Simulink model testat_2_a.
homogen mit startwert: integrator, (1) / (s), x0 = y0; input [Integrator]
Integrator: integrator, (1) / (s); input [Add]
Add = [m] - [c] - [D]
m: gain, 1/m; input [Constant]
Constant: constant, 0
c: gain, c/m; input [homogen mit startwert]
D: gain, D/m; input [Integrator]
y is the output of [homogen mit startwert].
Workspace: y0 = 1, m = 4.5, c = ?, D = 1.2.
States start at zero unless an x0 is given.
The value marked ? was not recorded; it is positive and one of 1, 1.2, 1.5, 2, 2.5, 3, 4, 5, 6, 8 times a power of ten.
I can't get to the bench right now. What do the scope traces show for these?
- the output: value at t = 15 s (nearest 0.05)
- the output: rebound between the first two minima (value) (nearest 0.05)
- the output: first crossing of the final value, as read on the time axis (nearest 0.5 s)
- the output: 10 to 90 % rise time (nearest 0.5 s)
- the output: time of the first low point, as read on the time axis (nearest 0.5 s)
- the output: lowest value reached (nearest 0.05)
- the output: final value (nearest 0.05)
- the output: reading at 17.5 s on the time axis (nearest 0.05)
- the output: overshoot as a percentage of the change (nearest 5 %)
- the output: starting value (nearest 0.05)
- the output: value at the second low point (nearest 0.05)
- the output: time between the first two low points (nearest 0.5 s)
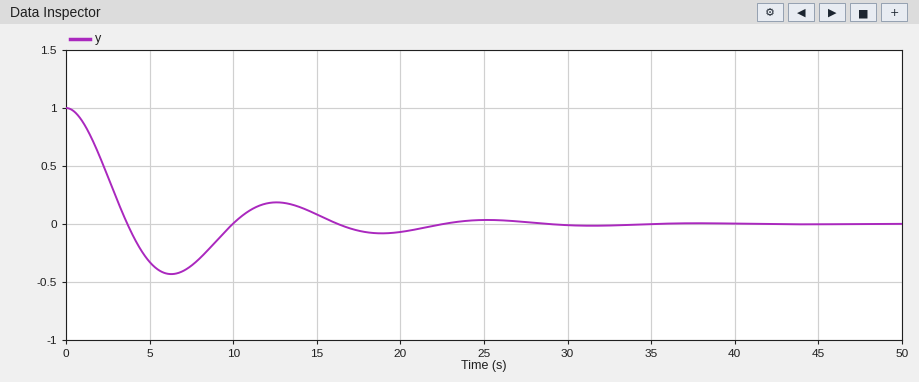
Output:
0.10
0.20
3.5 s
2.5 s
6.5 s
-0.45
0.00
-0.05
45 %
1.00
-0.10
12.5 s
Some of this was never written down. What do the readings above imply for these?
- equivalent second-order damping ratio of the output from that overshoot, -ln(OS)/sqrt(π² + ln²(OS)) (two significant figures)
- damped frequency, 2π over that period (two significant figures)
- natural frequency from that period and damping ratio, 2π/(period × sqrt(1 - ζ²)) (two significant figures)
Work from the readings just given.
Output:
0.25
0.50 rad/s
0.52 rad/s
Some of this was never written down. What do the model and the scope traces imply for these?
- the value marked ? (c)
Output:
1.2
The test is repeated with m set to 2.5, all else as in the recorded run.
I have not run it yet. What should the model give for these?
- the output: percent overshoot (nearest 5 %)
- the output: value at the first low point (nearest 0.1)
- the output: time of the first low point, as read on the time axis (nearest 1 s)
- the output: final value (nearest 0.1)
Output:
30 %
-0.3
5 s
0.0
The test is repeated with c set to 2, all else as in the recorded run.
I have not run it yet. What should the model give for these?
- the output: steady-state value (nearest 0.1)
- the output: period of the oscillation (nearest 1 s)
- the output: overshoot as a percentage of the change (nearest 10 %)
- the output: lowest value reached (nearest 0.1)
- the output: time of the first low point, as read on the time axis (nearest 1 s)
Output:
0.0
10 s
50 %
-0.5
5 s
